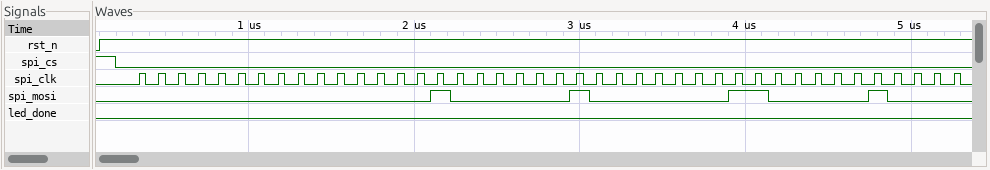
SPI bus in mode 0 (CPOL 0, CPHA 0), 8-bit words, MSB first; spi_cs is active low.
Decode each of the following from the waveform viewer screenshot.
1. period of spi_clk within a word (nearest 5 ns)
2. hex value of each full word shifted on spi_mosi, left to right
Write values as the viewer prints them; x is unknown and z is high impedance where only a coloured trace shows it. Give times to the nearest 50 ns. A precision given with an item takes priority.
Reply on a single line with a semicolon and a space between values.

120 ns; 00, 01, 02, 03, 04
